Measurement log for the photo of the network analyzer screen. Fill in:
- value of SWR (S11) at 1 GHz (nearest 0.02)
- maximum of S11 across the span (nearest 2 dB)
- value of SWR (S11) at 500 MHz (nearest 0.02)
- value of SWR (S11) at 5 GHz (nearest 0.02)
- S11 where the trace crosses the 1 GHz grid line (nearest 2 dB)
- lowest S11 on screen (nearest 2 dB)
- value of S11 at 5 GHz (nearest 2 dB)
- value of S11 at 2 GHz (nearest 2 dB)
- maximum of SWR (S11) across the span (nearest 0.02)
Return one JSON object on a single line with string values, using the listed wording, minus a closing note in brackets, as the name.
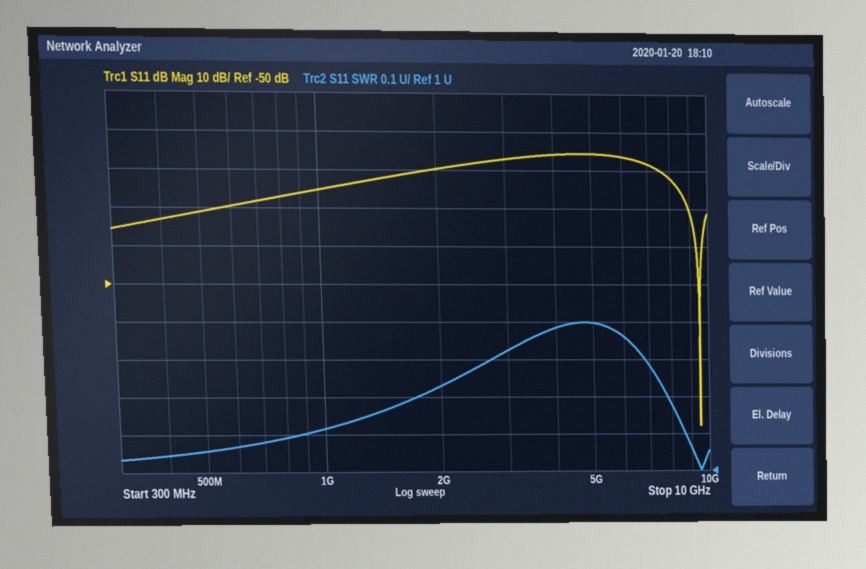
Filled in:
{"value of SWR (S11) at 1 GHz": "1.12", "maximum of S11 across the span": "-16 dB", "value of SWR (S11) at 500 MHz": "1.06", "value of SWR (S11) at 5 GHz": "1.40", "S11 where the trace crosses the 1 GHz grid line": "-26 dB", "lowest S11 on screen": "-88 dB", "value of S11 at 5 GHz": "-16 dB", "value of S11 at 2 GHz": "-20 dB", "maximum of SWR (S11) across the span": "1.40"}
